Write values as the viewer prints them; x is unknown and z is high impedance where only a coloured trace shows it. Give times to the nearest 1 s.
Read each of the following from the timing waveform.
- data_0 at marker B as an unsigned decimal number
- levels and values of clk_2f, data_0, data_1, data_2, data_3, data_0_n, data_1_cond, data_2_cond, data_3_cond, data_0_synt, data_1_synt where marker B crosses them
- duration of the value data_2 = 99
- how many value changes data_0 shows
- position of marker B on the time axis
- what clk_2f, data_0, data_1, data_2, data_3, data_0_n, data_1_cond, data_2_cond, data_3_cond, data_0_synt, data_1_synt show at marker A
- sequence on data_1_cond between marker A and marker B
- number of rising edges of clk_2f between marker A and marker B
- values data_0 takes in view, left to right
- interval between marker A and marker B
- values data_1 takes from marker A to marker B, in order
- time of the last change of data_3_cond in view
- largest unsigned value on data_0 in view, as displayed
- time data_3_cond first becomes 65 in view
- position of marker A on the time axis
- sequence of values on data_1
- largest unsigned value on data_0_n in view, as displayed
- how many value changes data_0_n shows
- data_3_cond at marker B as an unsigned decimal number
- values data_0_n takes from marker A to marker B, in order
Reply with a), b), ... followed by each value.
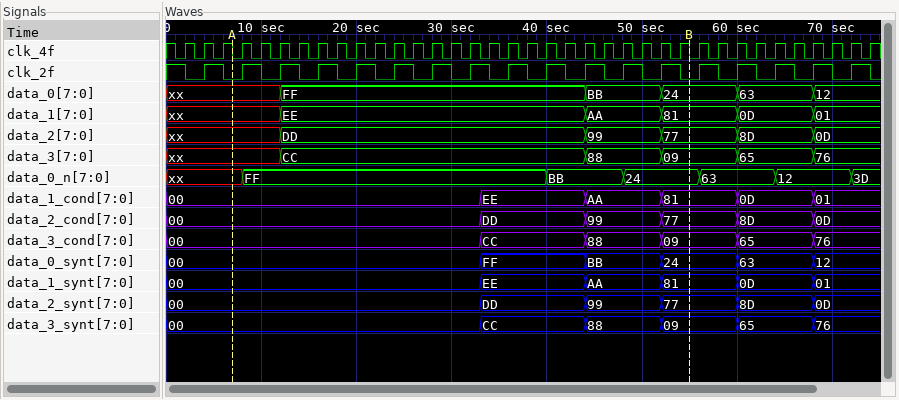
a) 36
b) clk_2f=0, data_0=24, data_1=81, data_2=77, data_3=09, data_0_n=24, data_1_cond=81, data_2_cond=77, data_3_cond=09, data_0_synt=24, data_1_synt=81
c) 8 s
d) 5
e) 55 s
f) clk_2f=0, data_0=xx, data_1=xx, data_2=xx, data_3=xx, data_0_n=xx, data_1_cond=00, data_2_cond=00, data_3_cond=00, data_0_synt=00, data_1_synt=00
g) 00, EE, AA, 81
h) 12
i) xx, FF, BB, 24, 63, 12
j) 48 s
k) xx, EE, AA, 81
l) 68 s
m) FF
n) 60 s
o) 7 s
p) xx, EE, AA, 81, 0D, 01
q) FF
r) 6
s) 9
t) xx, FF, BB, 24
